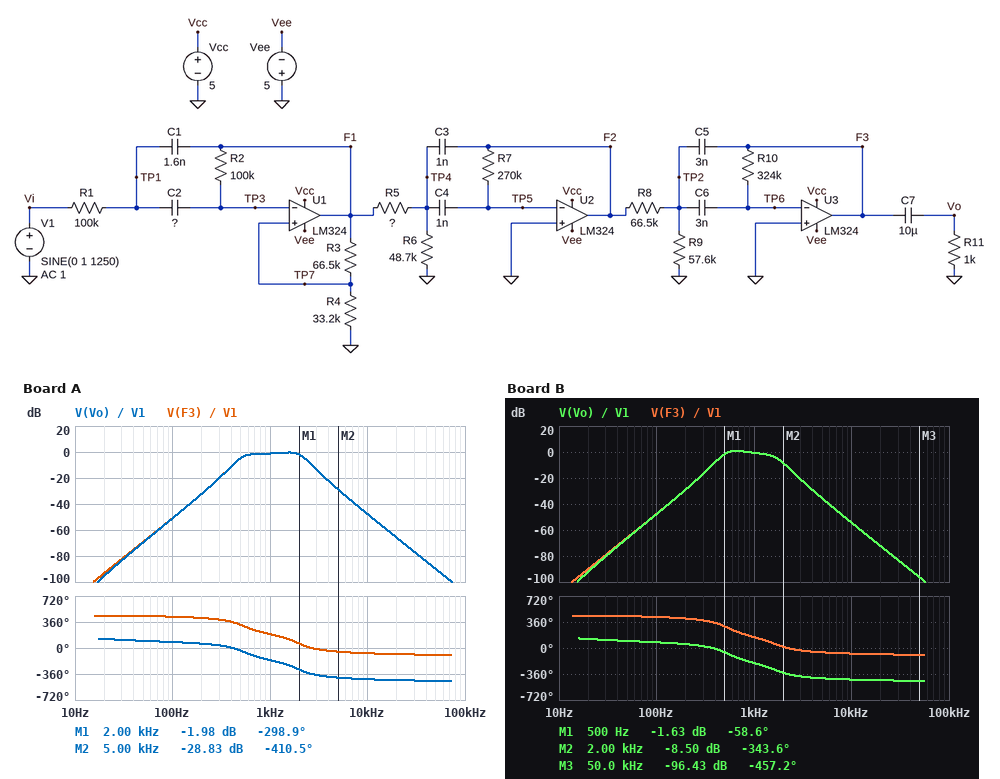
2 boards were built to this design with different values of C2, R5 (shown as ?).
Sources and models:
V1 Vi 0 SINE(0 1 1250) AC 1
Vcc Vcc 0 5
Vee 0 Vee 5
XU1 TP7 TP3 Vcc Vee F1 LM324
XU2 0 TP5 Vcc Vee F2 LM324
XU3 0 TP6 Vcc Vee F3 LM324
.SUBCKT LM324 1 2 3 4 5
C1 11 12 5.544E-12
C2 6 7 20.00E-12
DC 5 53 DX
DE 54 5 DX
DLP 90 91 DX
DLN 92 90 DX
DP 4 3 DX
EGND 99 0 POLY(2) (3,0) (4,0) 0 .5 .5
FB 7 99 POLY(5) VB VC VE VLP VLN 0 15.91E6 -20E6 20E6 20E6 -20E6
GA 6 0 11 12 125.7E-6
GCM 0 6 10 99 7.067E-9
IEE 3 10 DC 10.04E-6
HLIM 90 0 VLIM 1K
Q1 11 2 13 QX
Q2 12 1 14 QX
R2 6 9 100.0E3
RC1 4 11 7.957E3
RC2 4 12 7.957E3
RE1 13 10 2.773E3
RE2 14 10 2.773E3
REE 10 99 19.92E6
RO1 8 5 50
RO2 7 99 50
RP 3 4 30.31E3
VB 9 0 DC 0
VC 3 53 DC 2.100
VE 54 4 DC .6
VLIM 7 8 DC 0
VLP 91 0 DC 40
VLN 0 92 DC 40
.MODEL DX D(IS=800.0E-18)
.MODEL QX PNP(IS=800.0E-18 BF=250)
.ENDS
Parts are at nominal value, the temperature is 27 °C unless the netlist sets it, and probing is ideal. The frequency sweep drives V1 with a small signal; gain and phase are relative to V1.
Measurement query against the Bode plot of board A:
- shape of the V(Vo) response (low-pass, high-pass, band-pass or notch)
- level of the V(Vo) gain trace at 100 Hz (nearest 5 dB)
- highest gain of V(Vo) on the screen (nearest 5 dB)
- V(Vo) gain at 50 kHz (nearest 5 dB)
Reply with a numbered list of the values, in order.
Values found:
1. band-pass
2. -50 dB
3. 0 dB
4. -90 dB
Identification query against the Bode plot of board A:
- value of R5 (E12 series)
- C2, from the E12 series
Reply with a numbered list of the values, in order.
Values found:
1. 47 kΩ
2. 1.2 nF
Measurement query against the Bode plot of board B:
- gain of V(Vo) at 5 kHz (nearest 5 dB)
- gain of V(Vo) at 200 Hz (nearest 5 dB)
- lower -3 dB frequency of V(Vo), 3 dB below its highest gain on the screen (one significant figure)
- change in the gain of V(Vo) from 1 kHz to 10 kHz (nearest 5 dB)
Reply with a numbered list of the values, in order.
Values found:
1. -35 dB
2. -30 dB
3. 500 Hz
4. -55 dB
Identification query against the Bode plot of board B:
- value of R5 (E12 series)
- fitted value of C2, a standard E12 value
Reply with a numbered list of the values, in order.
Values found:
1. 100 kΩ
2. 2.7 nF
